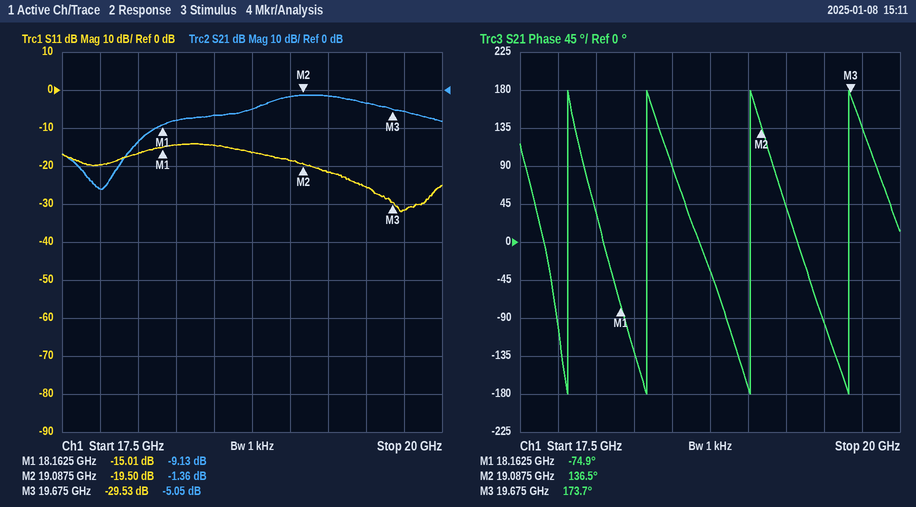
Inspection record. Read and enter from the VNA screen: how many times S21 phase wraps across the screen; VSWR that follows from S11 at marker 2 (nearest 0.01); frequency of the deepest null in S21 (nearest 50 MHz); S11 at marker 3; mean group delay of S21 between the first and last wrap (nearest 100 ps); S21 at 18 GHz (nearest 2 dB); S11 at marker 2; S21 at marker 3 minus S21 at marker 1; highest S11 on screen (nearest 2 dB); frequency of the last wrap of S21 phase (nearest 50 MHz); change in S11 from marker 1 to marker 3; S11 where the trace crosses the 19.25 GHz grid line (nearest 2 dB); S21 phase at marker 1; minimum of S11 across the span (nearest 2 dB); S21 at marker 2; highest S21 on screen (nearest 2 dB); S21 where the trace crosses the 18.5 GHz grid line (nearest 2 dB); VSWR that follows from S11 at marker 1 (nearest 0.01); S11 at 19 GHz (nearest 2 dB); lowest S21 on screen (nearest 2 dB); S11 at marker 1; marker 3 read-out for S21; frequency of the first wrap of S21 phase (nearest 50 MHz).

4
1.24
17.75 GHz
-29.53 dB
1.6 ns
-14 dB
-19.50 dB
4.08 dB
-14 dB
19.65 GHz
-14.52 dB
-22 dB
-74.9°
-32 dB
-1.36 dB
-2 dB
-6 dB
1.43
-18 dB
-26 dB
-15.01 dB
-5.05 dB
17.80 GHz
